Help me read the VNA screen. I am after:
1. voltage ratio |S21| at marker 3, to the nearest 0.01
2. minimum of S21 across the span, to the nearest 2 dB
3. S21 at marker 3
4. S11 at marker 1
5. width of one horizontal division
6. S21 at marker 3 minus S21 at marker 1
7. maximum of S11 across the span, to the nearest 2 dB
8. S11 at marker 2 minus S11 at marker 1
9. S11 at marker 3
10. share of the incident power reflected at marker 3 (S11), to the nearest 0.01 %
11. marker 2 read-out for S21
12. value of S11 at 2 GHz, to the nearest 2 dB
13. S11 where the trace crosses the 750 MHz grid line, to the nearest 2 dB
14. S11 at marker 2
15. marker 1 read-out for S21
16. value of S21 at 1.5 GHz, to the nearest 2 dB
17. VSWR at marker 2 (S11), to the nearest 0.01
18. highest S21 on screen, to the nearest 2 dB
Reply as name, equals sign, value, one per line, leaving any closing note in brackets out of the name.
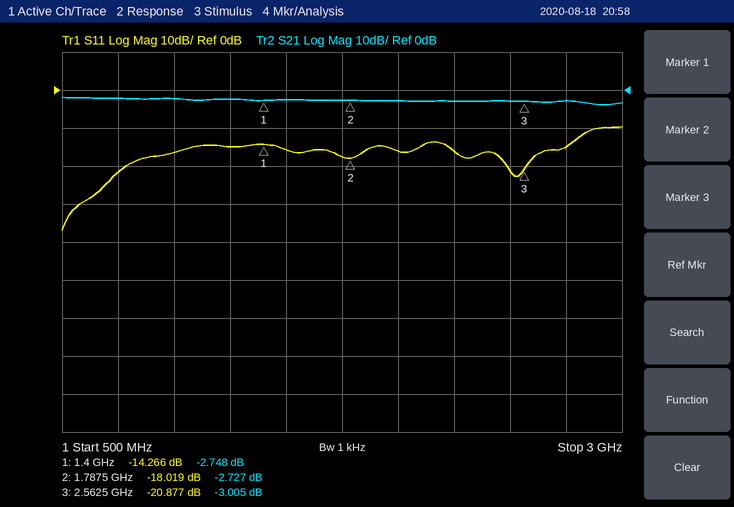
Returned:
voltage ratio |S21| at marker 3, to the nearest 0.01 = 0.71
minimum of S21 across the span, to the nearest 2 dB = -4 dB
S21 at marker 3 = -3.005 dB
S11 at marker 1 = -14.266 dB
width of one horizontal division = 250 MHz
S21 at marker 3 minus S21 at marker 1 = -0.257 dB
maximum of S11 across the span, to the nearest 2 dB = -10 dB
S11 at marker 2 minus S11 at marker 1 = -3.753 dB
S11 at marker 3 = -20.877 dB
share of the incident power reflected at marker 3 (S11), to the nearest 0.01 % = 0.82 %
marker 2 read-out for S21 = -2.727 dB
value of S11 at 2 GHz, to the nearest 2 dB = -16 dB
S11 where the trace crosses the 750 MHz grid line, to the nearest 2 dB = -22 dB
S11 at marker 2 = -18.019 dB
marker 1 read-out for S21 = -2.748 dB
value of S21 at 1.5 GHz, to the nearest 2 dB = -2 dB
VSWR at marker 2 (S11), to the nearest 0.01 = 1.29
highest S21 on screen, to the nearest 2 dB = -2 dB
